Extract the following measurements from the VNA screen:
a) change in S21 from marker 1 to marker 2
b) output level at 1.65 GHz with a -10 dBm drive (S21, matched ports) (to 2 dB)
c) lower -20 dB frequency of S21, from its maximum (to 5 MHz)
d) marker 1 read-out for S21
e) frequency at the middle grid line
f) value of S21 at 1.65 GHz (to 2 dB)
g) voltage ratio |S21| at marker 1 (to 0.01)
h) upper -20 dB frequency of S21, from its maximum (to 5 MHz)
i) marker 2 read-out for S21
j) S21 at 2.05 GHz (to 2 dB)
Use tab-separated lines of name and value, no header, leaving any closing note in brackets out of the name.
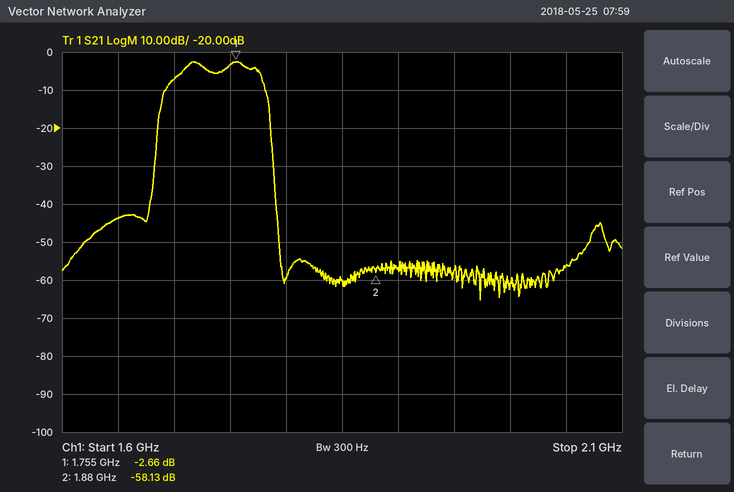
change in S21 from marker 1 to marker 2	-55.47 dB
output level at 1.65 GHz with a -10 dBm drive (S21, matched ports)	-54 dBm
lower -20 dB frequency of S21, from its maximum	1.685 GHz
marker 1 read-out for S21	-2.66 dB
frequency at the middle grid line	1.85 GHz
value of S21 at 1.65 GHz	-44 dB
voltage ratio |S21| at marker 1	0.74
upper -20 dB frequency of S21, from its maximum	1.785 GHz
marker 2 read-out for S21	-58.13 dB
S21 at 2.05 GHz	-56 dB
